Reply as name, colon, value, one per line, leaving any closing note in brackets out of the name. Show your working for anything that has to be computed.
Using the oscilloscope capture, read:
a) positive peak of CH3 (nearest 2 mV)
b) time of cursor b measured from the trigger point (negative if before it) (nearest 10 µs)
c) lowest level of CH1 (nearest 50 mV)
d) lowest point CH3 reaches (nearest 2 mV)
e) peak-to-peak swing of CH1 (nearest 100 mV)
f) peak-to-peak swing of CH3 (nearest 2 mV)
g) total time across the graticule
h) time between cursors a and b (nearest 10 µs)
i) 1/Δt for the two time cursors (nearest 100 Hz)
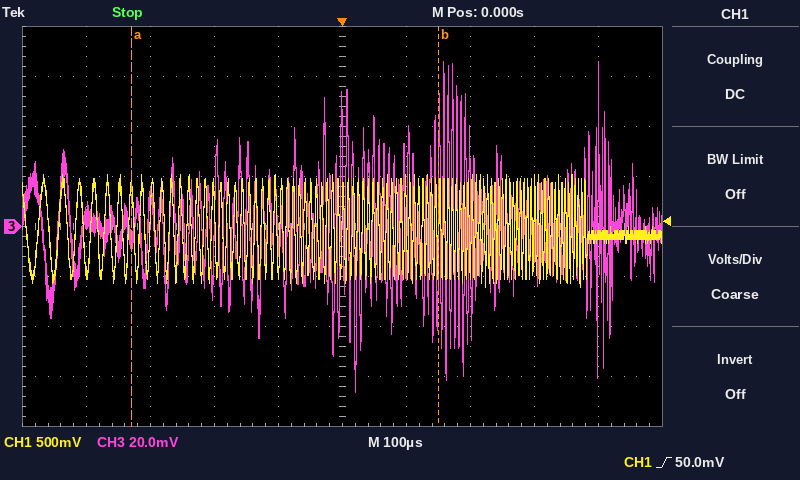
positive peak of CH3: 66 mV
time of cursor b measured from the trigger point (negative if before it): +150 µs
lowest level of CH1: -600 mV
lowest point CH3 reaches: -66 mV
peak-to-peak swing of CH1: 1.10 V
peak-to-peak swing of CH3: 66 mV − (-66 mV) = 132 mV
total time across the graticule: 1 ms
time between cursors a and b: 480 µs
1/Δt for the two time cursors: 1 / 480 µs ≈ 2.1 kHz
